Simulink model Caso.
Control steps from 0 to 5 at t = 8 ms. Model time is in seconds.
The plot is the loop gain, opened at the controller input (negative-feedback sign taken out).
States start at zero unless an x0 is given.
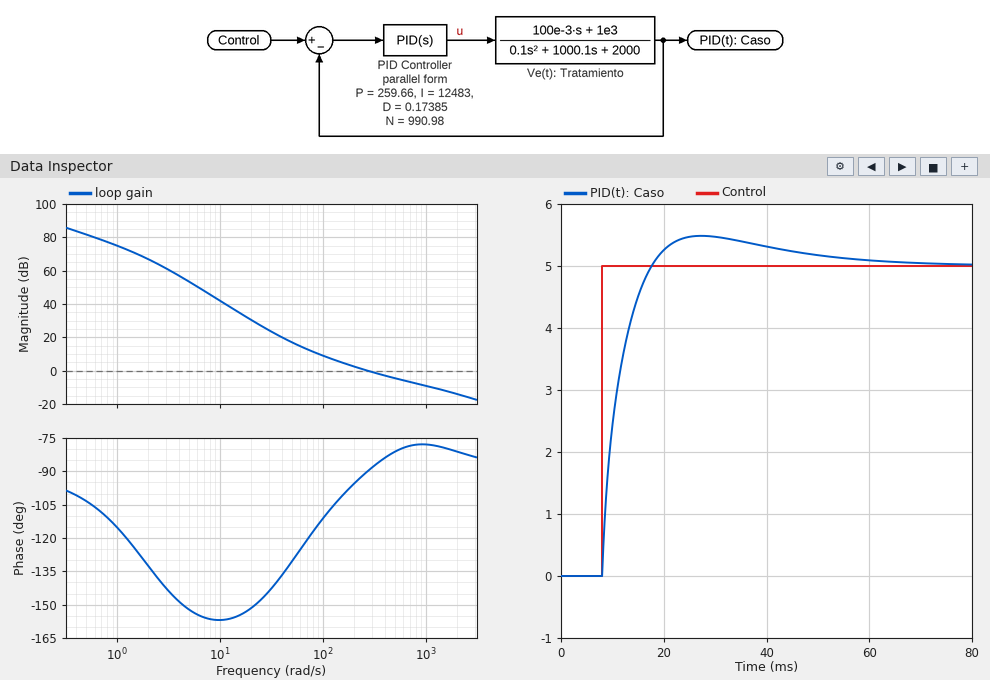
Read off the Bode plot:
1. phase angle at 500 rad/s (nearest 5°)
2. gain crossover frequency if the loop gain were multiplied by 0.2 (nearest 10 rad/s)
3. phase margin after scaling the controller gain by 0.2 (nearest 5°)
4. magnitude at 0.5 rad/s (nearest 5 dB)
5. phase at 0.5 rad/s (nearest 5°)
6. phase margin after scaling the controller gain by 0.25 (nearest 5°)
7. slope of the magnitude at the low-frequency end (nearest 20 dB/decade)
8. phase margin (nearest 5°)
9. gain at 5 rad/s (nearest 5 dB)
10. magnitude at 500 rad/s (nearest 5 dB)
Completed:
-80°
60 rad/s
55°
80 dB
-105°
60°
-20 dB/decade
90°
55 dB
-5 dB
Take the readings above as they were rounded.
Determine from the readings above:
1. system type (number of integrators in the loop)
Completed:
1
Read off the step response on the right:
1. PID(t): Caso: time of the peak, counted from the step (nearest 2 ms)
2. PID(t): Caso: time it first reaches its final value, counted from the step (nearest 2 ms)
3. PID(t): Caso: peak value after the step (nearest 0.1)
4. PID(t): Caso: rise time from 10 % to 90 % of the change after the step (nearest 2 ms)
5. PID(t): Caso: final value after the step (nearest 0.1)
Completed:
20 ms
10 ms
5.5
6 ms
5.0
